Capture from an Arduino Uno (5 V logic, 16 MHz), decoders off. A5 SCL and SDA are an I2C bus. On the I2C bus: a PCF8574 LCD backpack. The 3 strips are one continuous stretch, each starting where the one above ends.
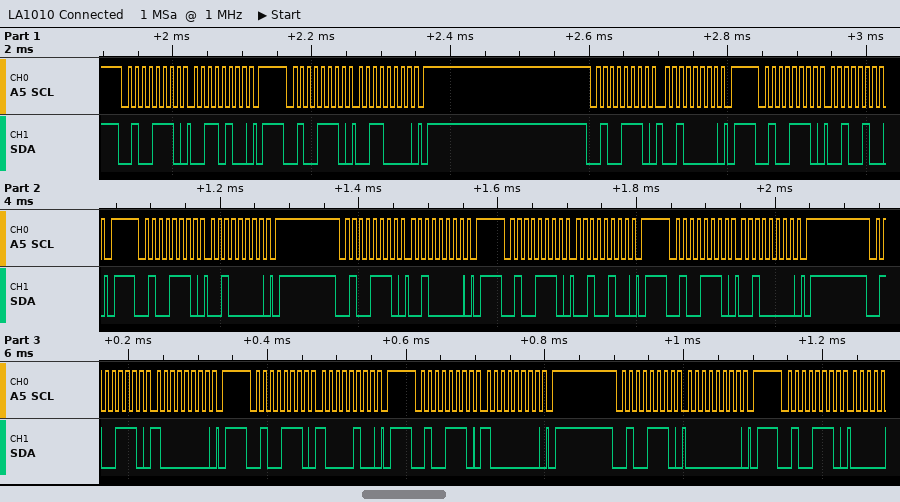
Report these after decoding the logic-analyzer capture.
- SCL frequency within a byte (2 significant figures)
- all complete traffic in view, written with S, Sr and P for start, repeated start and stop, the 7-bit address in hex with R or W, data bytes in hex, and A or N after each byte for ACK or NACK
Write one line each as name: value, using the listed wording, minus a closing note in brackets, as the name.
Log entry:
SCL frequency within a byte: 100 kHz
all complete traffic in view, written with S, Sr and P for start, repeated start and stop, the 7-bit address in hex with R or W, data bytes in hex, and A or N after each byte for ACK or NACK: S 27W A 34 A P S 27W A 30 A P S 27W A 20 A P S 27W A 24 A P S 27W A 20 A P S 27W A 20 A P S 27W A 24 A P S 27W A 20 A P S 27W A 80 A P S 27W A 84 A P S 27W A 80 A P S 27W A 00 A P S 27W A
